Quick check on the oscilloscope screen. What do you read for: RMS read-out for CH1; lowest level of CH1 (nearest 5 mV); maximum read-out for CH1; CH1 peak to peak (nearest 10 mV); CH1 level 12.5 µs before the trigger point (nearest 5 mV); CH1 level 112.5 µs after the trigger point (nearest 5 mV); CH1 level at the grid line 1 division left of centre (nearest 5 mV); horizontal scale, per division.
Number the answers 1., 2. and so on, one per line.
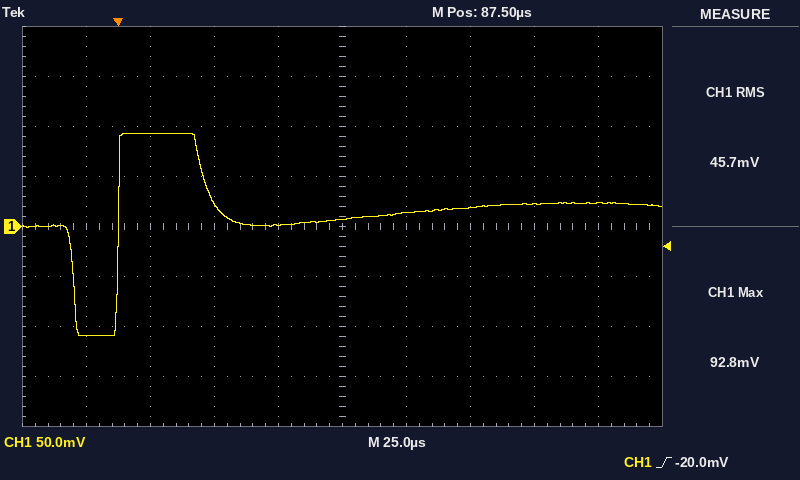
1. 45.7 mV
2. -110 mV
3. 92.8 mV
4. 200 mV
5. -110 mV
6. 15 mV
7. 0 mV
8. 25 µs
